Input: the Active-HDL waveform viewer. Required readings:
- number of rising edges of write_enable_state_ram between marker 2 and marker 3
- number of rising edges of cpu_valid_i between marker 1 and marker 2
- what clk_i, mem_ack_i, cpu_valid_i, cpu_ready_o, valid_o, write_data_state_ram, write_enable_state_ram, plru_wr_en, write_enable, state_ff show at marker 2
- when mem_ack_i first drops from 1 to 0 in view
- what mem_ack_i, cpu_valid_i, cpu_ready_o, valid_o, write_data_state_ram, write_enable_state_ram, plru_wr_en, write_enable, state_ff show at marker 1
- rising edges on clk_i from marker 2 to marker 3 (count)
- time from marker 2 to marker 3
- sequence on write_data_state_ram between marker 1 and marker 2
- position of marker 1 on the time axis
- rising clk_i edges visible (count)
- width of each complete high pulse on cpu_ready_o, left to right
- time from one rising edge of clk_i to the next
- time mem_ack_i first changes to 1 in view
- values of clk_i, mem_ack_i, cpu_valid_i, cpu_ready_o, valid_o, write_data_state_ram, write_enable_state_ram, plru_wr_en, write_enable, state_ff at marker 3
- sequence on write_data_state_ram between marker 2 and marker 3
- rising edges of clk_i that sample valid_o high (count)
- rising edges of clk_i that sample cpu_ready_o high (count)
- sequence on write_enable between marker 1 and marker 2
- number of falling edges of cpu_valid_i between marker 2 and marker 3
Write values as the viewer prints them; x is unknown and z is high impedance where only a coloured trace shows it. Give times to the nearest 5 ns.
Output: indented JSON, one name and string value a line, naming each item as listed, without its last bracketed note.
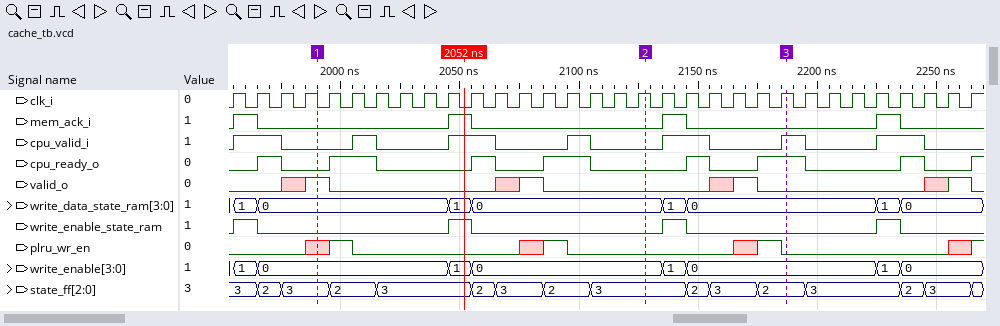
{
  "number of rising edges of write_enable_state_ram between marker 2 and marker 3": "1",
  "number of rising edges of cpu_valid_i between marker 1 and marker 2": "3",
  "what clk_i, mem_ack_i, cpu_valid_i, cpu_ready_o, valid_o, write_data_state_ram, write_enable_state_ram, plru_wr_en, write_enable, state_ff show at marker 2": "clk_i=1, mem_ack_i=0, cpu_valid_i=0, cpu_ready_o=0, valid_o=0, write_data_state_ram=0, write_enable_state_ram=0, plru_wr_en=0, write_enable=0, state_ff=3",
  "when mem_ack_i first drops from 1 to 0 in view": "1965 ns",
  "what mem_ack_i, cpu_valid_i, cpu_ready_o, valid_o, write_data_state_ram, write_enable_state_ram, plru_wr_en, write_enable, state_ff show at marker 1": "mem_ack_i=0, cpu_valid_i=0, cpu_ready_o=0, valid_o=1, write_data_state_ram=0, write_enable_state_ram=0, plru_wr_en=x, write_enable=0, state_ff=3",
  "rising edges on clk_i from marker 2 to marker 3": "6",
  "time from marker 2 to marker 3": "60 ns",
  "sequence on write_data_state_ram between marker 1 and marker 2": "0, 1, 0",
  "position of marker 1 on the time axis": "1990 ns",
  "rising clk_i edges visible": "32",
  "width of each complete high pulse on cpu_ready_o, left to right": "10 ns, 20 ns, 10 ns, 20 ns, 10 ns, 20 ns, 10 ns",
  "time from one rising edge of clk_i to the next": "10 ns",
  "time mem_ack_i first changes to 1 in view": "1955 ns",
  "values of clk_i, mem_ack_i, cpu_valid_i, cpu_ready_o, valid_o, write_data_state_ram, write_enable_state_ram, plru_wr_en, write_enable, state_ff at marker 3": "clk_i=1, mem_ack_i=0, cpu_valid_i=1, cpu_ready_o=1, valid_o=0, write_data_state_ram=0, write_enable_state_ram=0, plru_wr_en=0, write_enable=0, state_ff=2",
  "sequence on write_data_state_ram between marker 2 and marker 3": "0, 1, 0",
  "rising edges of clk_i that sample valid_o high": "4",
  "rising edges of clk_i that sample cpu_ready_o high": "10",
  "sequence on write_enable between marker 1 and marker 2": "0, 1, 0",
  "number of falling edges of cpu_valid_i between marker 2 and marker 3": "1"
}
